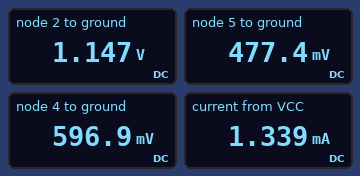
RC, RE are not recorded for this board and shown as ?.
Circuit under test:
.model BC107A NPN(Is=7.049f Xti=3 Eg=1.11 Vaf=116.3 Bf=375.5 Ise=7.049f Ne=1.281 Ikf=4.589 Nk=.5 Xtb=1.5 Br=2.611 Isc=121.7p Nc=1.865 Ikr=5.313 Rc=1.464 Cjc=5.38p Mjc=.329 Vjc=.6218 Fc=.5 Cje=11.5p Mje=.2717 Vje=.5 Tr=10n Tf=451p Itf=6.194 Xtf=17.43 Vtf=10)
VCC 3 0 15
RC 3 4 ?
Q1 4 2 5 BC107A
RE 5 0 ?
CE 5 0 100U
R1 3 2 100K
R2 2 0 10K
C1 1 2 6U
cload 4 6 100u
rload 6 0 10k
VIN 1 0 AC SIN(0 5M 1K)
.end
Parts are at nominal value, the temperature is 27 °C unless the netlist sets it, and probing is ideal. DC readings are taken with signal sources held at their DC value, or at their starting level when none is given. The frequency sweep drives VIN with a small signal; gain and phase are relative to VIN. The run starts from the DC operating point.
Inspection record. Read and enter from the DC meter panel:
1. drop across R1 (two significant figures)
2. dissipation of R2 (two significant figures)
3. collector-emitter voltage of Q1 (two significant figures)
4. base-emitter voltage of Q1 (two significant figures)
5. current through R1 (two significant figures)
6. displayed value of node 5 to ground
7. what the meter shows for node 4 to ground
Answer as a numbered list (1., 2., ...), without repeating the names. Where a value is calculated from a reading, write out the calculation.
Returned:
1. 15 V - 1.147 V = 14 V
2. (1.147 V)^2 / 10 kΩ = 130 µW
3. 596.9 mV - 477.4 mV = 120 mV
4. 1.147 V - 477.4 mV = 670 mV
5. (15 V - 1.147 V) / 100 kΩ = 140 µA
6. 477.4 mV
7. 596.9 mV
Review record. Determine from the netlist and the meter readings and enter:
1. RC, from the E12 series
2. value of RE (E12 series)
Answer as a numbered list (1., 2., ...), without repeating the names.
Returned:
1. 12 kΩ
2. 390 Ω
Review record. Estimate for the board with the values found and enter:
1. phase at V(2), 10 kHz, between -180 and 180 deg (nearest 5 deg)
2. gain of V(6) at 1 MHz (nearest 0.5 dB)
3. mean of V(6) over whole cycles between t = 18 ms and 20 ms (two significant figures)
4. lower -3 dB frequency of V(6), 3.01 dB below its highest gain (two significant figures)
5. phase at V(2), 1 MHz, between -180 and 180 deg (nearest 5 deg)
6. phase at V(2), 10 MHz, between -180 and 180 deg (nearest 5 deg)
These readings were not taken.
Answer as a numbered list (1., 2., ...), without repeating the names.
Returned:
1. 5 deg
2. 32.5 dB
3. 440 mV
4. 530 Hz
5. 0 deg
6. 0 deg
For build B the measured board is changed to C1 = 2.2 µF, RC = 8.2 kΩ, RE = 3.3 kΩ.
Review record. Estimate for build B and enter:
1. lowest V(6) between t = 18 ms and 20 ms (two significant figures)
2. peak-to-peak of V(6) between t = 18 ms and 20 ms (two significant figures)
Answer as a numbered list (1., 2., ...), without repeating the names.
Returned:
1. -200 mV
2. 380 mV
